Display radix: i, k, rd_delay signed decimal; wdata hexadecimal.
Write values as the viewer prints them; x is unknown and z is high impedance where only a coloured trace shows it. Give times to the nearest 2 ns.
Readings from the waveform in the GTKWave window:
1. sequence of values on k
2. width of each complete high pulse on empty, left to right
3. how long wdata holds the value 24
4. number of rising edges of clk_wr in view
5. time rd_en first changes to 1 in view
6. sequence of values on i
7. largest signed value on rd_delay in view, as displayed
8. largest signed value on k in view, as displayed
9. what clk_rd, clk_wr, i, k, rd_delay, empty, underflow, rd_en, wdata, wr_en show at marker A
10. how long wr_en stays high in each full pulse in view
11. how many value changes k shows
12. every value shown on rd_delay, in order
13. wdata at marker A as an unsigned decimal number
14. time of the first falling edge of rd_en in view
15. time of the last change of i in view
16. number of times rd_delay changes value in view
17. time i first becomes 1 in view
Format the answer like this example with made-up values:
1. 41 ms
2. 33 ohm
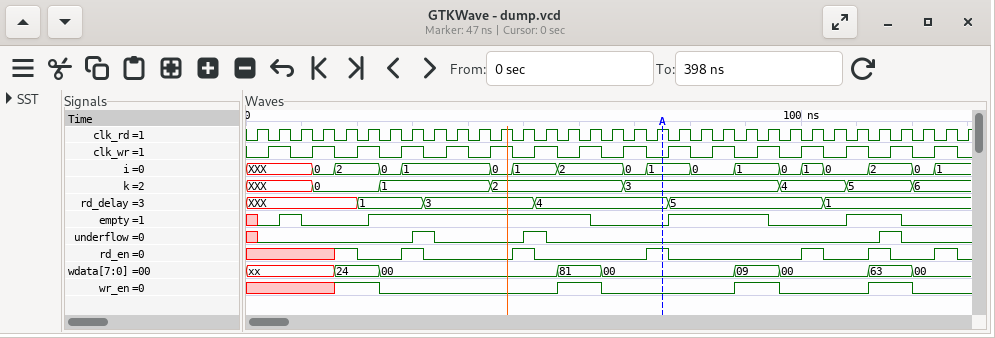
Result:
1. XXX, 0, 1, 2, 3, 4, 5, 6
2. 4 ns, 40 ns, 18 ns, 10 ns
3. 8 ns
4. 16
5. 16 ns
6. XXX, 0, 2, 0, 1, 0, 1, 2, 0, 1, 0, 1, 0, 1, 0, 2, 0, 1
7. 5
8. 6
9. clk_rd=1, clk_wr=0, i=1, k=3, rd_delay=4, empty=0, underflow=0, rd_en=1, wdata=00, wr_en=0
10. 8 ns, 8 ns, 8 ns
11. 7
12. XXX, 1, 3, 4, 5, 1
13. 0
14. 20 ns
15. 124 ns
16. 5
17. 28 ns
